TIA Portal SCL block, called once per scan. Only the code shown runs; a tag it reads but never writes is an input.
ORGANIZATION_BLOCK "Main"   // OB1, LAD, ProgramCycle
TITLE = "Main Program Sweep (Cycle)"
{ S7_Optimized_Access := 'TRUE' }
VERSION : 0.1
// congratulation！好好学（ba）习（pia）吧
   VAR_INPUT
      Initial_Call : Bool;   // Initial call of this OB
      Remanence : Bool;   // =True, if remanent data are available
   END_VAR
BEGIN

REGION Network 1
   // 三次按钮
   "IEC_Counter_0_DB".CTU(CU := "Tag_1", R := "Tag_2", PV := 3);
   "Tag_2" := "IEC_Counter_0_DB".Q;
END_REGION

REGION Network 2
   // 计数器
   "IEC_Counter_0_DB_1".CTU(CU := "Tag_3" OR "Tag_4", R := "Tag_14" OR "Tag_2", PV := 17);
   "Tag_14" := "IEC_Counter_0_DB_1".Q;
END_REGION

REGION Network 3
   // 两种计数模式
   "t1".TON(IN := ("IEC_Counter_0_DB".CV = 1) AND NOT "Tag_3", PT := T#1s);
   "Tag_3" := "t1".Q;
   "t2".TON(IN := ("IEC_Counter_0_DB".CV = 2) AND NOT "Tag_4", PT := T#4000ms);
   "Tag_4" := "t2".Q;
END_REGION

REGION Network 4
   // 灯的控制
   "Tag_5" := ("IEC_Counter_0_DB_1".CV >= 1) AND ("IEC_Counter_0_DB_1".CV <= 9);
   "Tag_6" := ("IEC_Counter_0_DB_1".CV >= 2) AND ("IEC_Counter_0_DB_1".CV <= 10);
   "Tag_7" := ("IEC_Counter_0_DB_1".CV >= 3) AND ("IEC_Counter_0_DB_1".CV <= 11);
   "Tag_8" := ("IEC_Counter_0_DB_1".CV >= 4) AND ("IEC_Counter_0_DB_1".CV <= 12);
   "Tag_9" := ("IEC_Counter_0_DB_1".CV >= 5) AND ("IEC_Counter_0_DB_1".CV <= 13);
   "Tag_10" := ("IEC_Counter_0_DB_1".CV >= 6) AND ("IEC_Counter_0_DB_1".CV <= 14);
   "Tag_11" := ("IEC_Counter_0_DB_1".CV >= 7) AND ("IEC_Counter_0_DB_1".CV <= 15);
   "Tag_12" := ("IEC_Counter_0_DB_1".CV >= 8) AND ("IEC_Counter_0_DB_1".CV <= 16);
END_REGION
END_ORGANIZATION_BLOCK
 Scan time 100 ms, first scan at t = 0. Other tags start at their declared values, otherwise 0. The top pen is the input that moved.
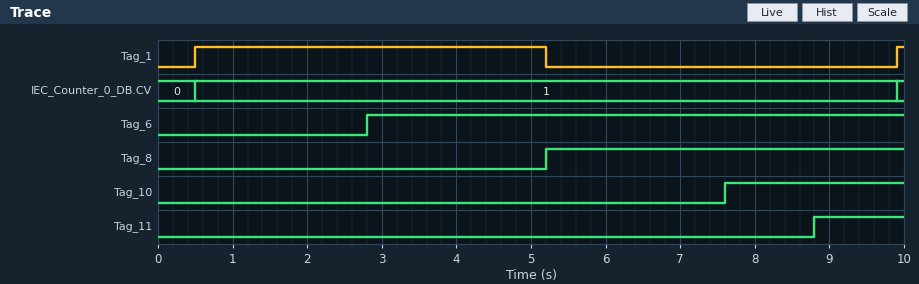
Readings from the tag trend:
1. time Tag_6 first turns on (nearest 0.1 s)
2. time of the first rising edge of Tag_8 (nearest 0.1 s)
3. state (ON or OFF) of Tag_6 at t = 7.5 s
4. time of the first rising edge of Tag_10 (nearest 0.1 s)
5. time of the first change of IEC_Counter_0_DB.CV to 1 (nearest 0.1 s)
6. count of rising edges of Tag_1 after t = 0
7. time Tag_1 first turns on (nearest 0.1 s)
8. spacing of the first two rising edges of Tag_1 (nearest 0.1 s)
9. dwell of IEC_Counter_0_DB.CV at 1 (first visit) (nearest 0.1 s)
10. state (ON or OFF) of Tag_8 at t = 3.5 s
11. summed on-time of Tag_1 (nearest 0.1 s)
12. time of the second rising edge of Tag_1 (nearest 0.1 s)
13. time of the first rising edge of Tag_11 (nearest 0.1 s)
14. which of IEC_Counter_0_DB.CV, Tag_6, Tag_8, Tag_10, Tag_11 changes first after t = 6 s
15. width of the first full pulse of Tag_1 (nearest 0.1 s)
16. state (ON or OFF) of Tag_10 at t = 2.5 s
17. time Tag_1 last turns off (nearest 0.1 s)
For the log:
2.8 s
5.2 s
ON
7.6 s
0.5 s
2
0.5 s
9.4 s
9.4 s
OFF
4.8 s
9.9 s
8.8 s
Tag_10
4.7 s
OFF
5.2 s
